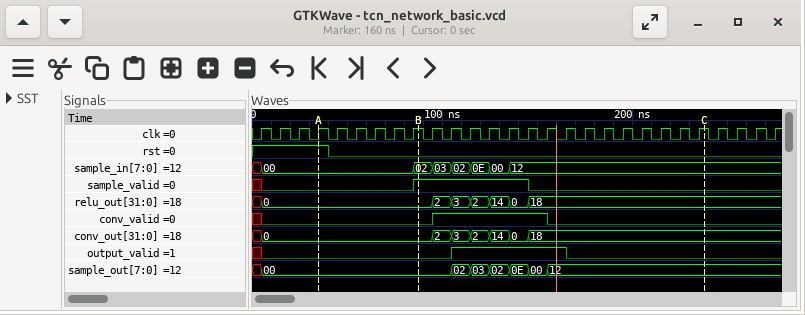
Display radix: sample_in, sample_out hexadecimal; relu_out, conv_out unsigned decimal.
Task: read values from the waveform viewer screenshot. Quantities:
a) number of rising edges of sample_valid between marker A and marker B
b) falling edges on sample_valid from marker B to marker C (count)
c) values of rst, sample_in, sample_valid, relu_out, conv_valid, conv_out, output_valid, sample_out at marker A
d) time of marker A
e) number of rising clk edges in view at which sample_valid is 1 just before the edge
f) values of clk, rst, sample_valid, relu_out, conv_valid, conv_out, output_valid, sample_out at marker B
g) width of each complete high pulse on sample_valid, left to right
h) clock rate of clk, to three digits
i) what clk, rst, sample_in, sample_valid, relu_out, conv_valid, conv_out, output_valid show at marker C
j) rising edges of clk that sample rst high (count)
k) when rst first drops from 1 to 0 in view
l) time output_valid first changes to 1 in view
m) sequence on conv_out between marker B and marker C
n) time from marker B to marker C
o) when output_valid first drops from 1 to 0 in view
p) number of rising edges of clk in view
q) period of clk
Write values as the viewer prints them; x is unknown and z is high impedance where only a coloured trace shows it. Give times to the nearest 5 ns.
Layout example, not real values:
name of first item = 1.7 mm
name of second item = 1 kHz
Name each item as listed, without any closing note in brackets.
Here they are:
number of rising edges of sample_valid between marker A and marker B = 1
falling edges on sample_valid from marker B to marker C = 1
values of rst, sample_in, sample_valid, relu_out, conv_valid, conv_out, output_valid, sample_out at marker A = rst=1, sample_in=00, sample_valid=0, relu_out=0, conv_valid=0, conv_out=0, output_valid=0, sample_out=00
time of marker A = 35 ns
number of rising clk edges in view at which sample_valid is 1 just before the edge = 6
values of clk, rst, sample_valid, relu_out, conv_valid, conv_out, output_valid, sample_out at marker B = clk=1, rst=0, sample_valid=1, relu_out=0, conv_valid=0, conv_out=0, output_valid=0, sample_out=00
width of each complete high pulse on sample_valid, left to right = 60 ns
clock rate of clk, to three digits = 100 MHz
what clk, rst, sample_in, sample_valid, relu_out, conv_valid, conv_out, output_valid show at marker C = clk=1, rst=0, sample_in=12, sample_valid=0, relu_out=18, conv_valid=0, conv_out=18, output_valid=0
rising edges of clk that sample rst high = 4
when rst first drops from 1 to 0 in view = 40 ns
time output_valid first changes to 1 in view = 105 ns
sequence on conv_out between marker B and marker C = 0, 2, 3, 2, 14, 0, 18
time from marker B to marker C = 150 ns
when output_valid first drops from 1 to 0 in view = 165 ns
number of rising edges of clk in view = 28
period of clk = 10 ns
